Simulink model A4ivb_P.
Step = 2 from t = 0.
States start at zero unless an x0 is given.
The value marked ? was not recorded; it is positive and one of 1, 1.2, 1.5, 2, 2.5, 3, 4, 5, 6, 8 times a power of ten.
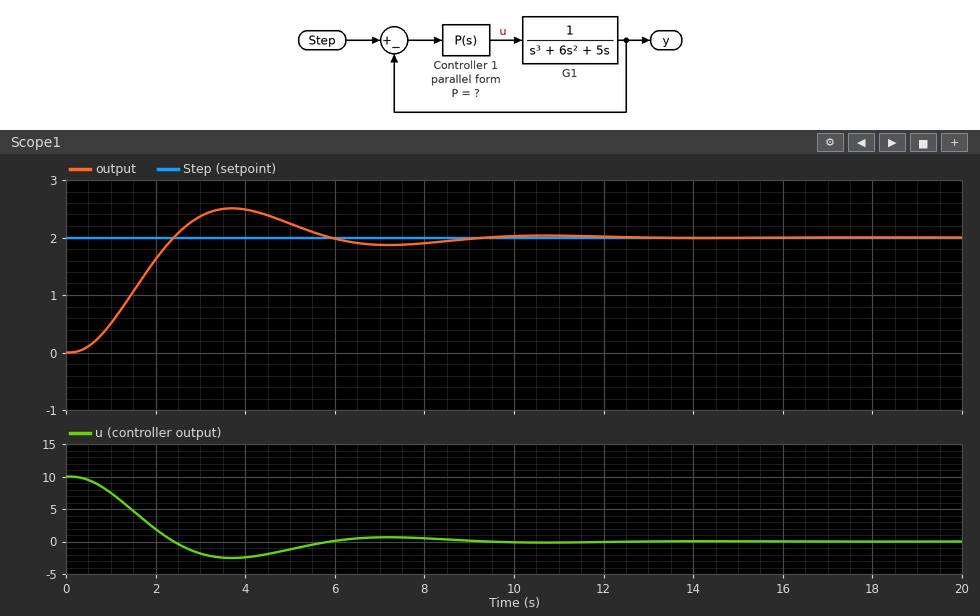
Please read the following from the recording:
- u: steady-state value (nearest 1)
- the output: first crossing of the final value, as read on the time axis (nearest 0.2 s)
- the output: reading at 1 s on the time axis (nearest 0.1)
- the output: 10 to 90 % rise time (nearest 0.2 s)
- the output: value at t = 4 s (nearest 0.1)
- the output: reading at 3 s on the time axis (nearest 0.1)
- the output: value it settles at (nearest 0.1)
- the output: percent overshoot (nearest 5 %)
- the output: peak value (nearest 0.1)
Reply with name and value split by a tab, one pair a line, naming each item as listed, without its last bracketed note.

u: steady-state value	0
the output: first crossing of the final value, as read on the time axis	2.4 s
the output: reading at 1 s on the time axis	0.5
the output: 10 to 90 % rise time	1.6 s
the output: value at t = 4 s	2.5
the output: reading at 3 s on the time axis	2.4
the output: value it settles at	2.0
the output: percent overshoot	25 %
the output: peak value	2.5
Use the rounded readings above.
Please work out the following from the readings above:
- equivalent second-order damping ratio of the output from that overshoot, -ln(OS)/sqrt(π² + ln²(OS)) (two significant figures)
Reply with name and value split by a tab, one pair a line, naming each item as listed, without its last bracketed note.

equivalent second-order damping ratio of the output from that overshoot, -ln(OS)/sqrt(π² + ln²(OS))	0.40
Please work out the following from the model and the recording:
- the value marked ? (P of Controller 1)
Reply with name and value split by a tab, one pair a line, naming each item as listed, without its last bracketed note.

the value marked ?	5
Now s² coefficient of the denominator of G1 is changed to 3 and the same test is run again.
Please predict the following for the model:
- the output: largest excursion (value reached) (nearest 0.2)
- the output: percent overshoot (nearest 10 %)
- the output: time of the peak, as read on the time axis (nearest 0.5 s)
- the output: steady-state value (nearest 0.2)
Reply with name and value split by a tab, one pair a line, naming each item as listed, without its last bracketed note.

the output: largest excursion (value reached)	2.4
the output: percent overshoot	20 %
the output: time of the peak, as read on the time axis	2.5 s
the output: steady-state value	2.0
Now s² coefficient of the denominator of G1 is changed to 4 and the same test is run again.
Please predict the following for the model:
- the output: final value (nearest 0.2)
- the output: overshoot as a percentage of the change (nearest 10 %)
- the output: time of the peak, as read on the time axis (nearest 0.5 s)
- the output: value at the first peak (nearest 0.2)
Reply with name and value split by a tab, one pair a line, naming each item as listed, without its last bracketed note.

the output: final value	2.0
the output: overshoot as a percentage of the change	20 %
the output: time of the peak, as read on the time axis	3.0 s
the output: value at the first peak	2.4
